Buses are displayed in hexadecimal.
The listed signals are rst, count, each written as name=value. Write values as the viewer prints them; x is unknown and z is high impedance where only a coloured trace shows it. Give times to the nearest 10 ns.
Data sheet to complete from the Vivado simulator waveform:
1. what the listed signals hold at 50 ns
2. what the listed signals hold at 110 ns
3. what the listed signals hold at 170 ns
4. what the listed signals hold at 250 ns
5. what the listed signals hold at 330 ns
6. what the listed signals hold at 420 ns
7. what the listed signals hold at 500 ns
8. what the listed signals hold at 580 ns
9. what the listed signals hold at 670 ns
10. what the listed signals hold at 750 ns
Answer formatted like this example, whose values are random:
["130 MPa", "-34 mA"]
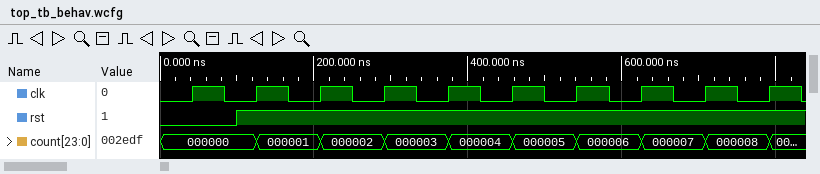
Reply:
["rst=0, count=000000", "rst=1, count=000000", "rst=1, count=000001", "rst=1, count=000002", "rst=1, count=000003", "rst=1, count=000004", "rst=1, count=000005", "rst=1, count=000006", "rst=1, count=000007", "rst=1, count=000008"]
